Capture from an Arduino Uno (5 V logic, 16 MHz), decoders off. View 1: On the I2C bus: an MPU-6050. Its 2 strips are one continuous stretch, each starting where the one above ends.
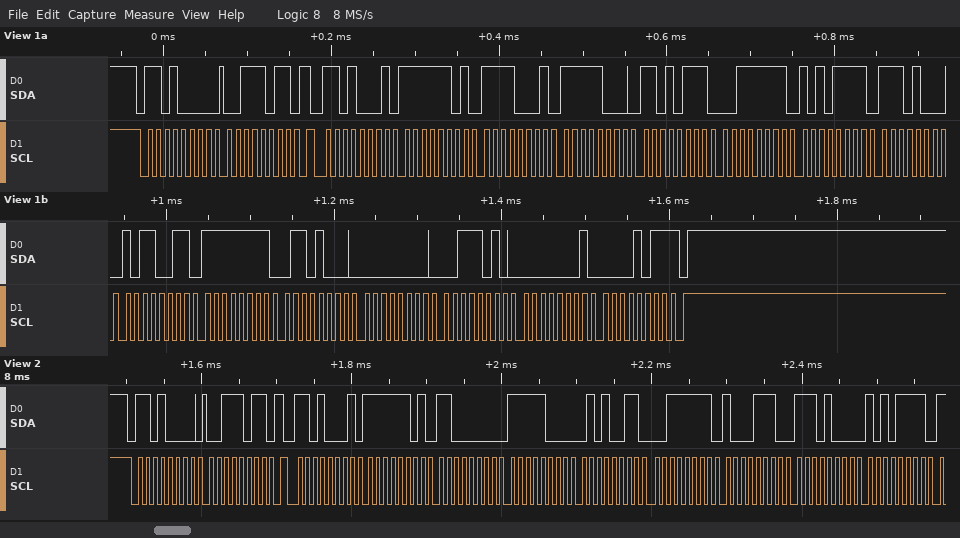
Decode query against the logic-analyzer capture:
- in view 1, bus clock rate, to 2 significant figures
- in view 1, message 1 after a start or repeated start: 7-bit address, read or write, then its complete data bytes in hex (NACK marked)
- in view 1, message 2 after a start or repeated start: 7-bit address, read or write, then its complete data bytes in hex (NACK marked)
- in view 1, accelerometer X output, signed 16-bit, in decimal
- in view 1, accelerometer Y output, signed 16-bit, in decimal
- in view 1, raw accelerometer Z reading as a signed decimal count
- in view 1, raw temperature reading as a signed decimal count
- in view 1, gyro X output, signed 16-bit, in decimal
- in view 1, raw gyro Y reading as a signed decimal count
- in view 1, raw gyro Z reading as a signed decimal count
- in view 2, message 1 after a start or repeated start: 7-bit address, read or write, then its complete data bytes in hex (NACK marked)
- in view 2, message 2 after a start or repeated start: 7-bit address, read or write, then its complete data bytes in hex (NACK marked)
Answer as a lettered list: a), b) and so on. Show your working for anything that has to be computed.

a) 100 kHz
b) 0x68 write: 3B
c) 0x68 read: FD F1 F8 D7 3F AF E8 B3 FF 68 00 3A 01 0B NACK
d) 0xFDF1 = -527
e) 0xF8D7 = -1833
f) 0x3FAF = 16303
g) 0xE8B3 = -5965
h) 0xFF68 = -152
i) 0x003A = 58
j) 0x010B = 267
k) 0x68 write: 3B
l) 0x68 read: FD C0 F8 53 3F 8E E8 AF
